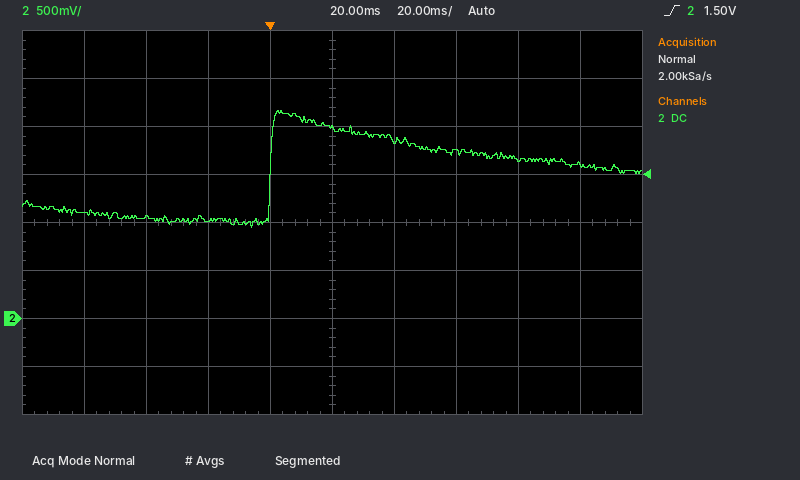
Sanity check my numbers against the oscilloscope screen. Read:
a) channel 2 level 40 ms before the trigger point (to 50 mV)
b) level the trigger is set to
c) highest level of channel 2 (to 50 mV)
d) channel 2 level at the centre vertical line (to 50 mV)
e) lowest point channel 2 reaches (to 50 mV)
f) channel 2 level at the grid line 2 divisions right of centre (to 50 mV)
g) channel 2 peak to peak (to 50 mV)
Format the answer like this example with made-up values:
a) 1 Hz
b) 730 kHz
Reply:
a) 1.05 V
b) 1.50 V
c) 2.15 V
d) 2.00 V
e) 950 mV
f) 1.75 V
g) 1.20 V
